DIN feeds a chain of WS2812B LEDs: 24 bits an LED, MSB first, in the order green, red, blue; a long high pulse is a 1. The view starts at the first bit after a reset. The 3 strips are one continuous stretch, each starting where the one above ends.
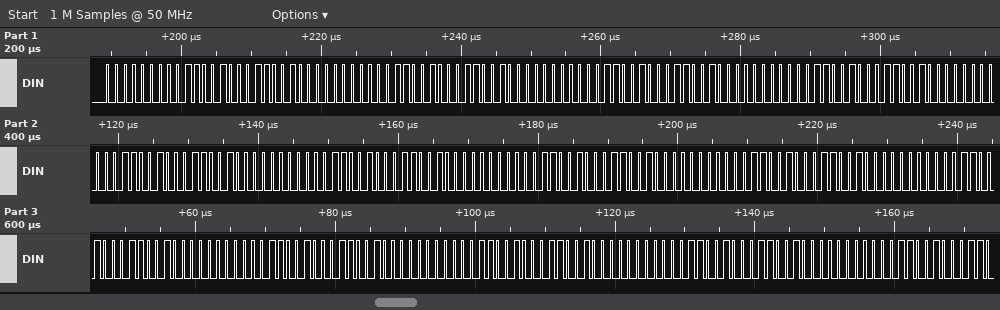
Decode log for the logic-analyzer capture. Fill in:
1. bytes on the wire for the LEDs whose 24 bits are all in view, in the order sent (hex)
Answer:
00 64 64 00 64 64 00 64 64 00 64 64 00 64 64 00 64 64 00 64 64 00 64 64 00 64 64 00 64 64 00 64 64 00 64 64
